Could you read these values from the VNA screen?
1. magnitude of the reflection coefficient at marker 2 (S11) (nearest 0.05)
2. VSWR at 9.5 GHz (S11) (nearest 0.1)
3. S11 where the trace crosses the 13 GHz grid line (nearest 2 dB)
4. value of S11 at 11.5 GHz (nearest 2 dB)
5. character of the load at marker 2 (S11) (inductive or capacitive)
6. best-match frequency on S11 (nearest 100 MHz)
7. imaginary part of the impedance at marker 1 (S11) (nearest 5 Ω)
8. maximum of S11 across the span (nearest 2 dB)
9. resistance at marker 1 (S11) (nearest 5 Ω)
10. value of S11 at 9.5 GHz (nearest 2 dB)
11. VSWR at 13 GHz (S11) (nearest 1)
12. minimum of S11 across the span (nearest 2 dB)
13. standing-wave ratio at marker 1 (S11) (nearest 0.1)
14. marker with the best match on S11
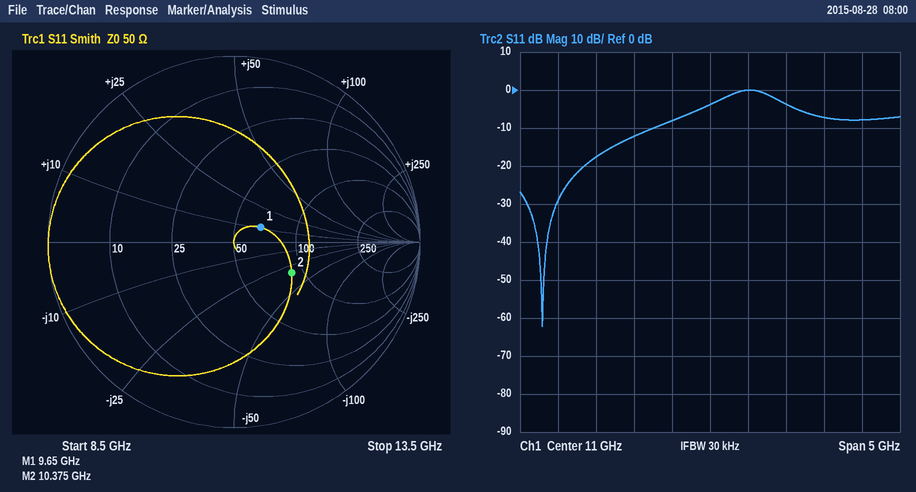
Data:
0.35
1.3
-8 dB
0 dB
capacitive
8.8 GHz
+10 Ω
0 dB
65 Ω
-18 dB
2
-62 dB
1.4
marker 1
